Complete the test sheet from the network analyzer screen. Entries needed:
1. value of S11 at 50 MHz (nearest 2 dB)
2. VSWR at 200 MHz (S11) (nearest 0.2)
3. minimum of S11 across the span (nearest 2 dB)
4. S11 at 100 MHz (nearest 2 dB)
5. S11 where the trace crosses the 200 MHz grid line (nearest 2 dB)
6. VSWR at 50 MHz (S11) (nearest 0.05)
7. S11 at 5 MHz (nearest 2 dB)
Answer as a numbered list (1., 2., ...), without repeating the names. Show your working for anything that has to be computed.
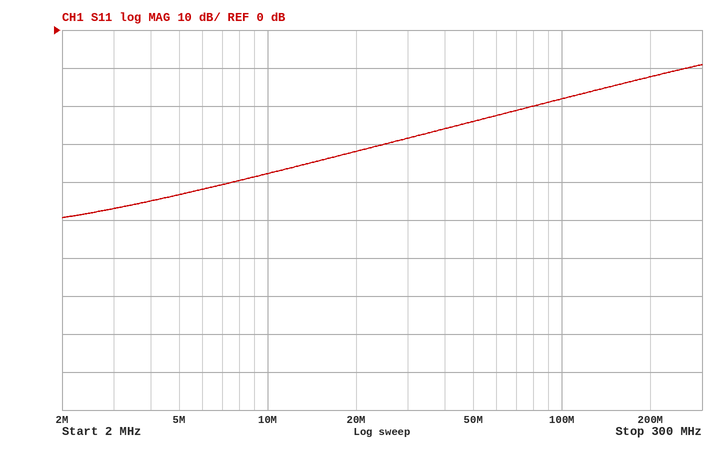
1. -24 dB
2. |Γ| = 10^(-12/20) = 0.2512; VSWR = (1 + 0.2512)/(1 − 0.2512) ≈ 1.67, so 1.6 to the nearest 0.2
3. -50 dB
4. -18 dB
5. -12 dB
6. |Γ| = 10^(-24/20) = 0.0631; VSWR = (1 + 0.0631)/(1 − 0.0631) ≈ 1.13, so 1.15 to the nearest 0.05
7. -44 dB
